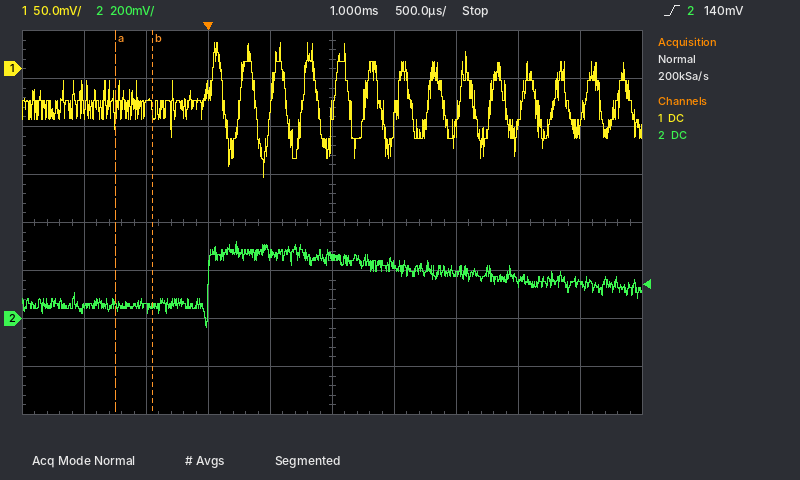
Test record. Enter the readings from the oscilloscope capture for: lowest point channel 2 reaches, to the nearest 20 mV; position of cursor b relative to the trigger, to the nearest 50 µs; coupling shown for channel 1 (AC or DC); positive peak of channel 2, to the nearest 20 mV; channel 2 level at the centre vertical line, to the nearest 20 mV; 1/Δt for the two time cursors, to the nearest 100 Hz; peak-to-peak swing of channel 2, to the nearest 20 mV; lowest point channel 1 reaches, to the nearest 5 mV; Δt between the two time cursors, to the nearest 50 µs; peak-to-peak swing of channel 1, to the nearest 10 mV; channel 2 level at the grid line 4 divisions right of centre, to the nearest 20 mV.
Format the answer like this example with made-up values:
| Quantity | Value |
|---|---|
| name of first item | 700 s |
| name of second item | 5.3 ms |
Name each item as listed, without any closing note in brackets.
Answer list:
| Quantity | Value |
|---|---|
| lowest point channel 2 reaches, to the nearest 20 mV | -40 mV |
| position of cursor b relative to the trigger, to the nearest 50 µs | -450 µs |
| coupling shown for channel 1 | DC |
| positive peak of channel 2, to the nearest 20 mV | 320 mV |
| channel 2 level at the centre vertical line, to the nearest 20 mV | 260 mV |
| 1/Δt for the two time cursors, to the nearest 100 Hz | 3.3 kHz |
| peak-to-peak swing of channel 2, to the nearest 20 mV | 360 mV |
| lowest point channel 1 reaches, to the nearest 5 mV | -115 mV |
| Δt between the two time cursors, to the nearest 50 µs | 300 µs |
| peak-to-peak swing of channel 1, to the nearest 10 mV | 140 mV |
| channel 2 level at the grid line 4 divisions right of centre, to the nearest 20 mV | 140 mV |
